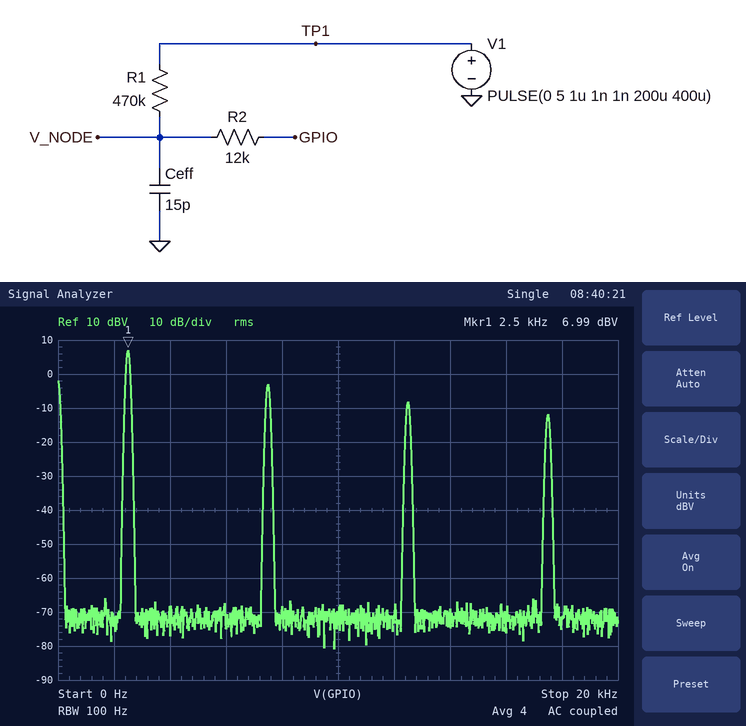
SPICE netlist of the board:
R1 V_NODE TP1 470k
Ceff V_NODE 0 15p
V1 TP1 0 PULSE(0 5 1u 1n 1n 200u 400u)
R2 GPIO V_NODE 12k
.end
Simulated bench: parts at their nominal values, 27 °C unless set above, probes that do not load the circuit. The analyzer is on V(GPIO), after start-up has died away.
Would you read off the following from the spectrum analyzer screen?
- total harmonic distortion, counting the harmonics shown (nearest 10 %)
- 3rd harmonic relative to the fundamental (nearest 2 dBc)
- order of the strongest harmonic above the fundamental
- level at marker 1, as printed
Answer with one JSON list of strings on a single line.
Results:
["40 %", "-10 dBc", "3", "6.99 dBV"]
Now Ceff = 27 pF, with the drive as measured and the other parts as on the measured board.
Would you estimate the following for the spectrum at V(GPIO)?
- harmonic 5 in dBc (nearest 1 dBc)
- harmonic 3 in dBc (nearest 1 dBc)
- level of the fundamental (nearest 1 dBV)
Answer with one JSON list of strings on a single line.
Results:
["-17 dBc", "-11 dBc", "7 dBV"]
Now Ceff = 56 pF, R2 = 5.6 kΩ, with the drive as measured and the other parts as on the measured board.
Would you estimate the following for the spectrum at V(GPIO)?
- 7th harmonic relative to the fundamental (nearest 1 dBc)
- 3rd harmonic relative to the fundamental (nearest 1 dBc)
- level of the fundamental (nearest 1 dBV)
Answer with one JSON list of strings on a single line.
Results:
["-26 dBc", "-13 dBc", "6 dBV"]
